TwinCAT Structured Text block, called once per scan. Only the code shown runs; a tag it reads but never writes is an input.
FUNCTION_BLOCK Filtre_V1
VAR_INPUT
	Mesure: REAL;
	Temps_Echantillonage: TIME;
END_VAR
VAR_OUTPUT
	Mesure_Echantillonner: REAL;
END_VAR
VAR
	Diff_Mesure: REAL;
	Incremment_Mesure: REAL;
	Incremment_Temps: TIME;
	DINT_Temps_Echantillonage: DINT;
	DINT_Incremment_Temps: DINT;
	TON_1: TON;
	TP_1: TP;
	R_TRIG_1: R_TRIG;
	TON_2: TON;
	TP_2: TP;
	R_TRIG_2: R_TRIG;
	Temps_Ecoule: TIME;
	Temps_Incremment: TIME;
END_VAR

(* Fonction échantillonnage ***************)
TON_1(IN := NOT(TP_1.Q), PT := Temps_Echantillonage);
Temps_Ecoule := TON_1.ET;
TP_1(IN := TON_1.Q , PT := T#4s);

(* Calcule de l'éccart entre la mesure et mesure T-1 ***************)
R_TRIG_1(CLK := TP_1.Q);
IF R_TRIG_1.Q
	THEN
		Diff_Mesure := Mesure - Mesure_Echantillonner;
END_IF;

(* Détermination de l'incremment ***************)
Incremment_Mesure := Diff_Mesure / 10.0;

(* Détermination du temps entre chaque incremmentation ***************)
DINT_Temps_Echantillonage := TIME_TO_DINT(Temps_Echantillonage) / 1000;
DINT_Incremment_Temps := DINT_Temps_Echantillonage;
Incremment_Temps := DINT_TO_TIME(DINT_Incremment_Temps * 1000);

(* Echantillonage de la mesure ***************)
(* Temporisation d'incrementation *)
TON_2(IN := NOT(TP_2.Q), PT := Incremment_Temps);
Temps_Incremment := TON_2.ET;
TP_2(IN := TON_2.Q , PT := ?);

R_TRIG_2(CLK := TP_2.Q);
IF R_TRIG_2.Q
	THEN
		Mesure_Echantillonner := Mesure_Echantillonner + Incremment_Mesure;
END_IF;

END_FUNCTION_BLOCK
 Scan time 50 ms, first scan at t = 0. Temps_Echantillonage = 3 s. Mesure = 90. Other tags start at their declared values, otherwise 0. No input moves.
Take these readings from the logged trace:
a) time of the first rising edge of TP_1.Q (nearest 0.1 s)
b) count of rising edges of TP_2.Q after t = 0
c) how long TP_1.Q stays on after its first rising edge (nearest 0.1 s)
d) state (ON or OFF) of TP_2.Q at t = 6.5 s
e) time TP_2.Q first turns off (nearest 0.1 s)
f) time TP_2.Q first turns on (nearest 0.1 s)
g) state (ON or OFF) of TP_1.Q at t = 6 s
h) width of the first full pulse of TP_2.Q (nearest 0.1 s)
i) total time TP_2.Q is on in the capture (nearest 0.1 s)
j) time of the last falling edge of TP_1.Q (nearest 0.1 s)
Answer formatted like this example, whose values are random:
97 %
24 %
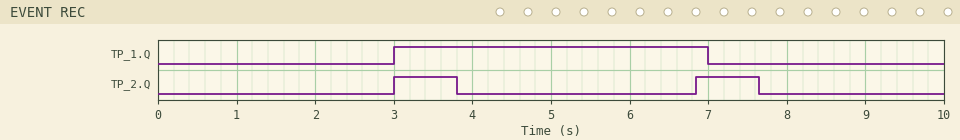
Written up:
3.0 s
2
4.0 s
OFF
3.8 s
3.0 s
ON
0.8 s
1.6 s
7.0 s
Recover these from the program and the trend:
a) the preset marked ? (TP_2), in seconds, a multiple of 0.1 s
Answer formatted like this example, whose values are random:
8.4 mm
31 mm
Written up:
0.8 s
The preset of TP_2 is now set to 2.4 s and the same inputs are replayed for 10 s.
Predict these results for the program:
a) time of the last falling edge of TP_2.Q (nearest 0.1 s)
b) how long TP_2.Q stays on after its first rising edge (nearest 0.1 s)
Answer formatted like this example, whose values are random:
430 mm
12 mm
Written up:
5.4 s
2.4 s
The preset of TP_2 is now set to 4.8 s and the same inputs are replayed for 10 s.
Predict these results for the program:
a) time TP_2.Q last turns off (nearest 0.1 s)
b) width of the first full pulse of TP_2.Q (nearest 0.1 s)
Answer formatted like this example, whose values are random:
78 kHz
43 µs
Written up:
7.8 s
4.8 s
